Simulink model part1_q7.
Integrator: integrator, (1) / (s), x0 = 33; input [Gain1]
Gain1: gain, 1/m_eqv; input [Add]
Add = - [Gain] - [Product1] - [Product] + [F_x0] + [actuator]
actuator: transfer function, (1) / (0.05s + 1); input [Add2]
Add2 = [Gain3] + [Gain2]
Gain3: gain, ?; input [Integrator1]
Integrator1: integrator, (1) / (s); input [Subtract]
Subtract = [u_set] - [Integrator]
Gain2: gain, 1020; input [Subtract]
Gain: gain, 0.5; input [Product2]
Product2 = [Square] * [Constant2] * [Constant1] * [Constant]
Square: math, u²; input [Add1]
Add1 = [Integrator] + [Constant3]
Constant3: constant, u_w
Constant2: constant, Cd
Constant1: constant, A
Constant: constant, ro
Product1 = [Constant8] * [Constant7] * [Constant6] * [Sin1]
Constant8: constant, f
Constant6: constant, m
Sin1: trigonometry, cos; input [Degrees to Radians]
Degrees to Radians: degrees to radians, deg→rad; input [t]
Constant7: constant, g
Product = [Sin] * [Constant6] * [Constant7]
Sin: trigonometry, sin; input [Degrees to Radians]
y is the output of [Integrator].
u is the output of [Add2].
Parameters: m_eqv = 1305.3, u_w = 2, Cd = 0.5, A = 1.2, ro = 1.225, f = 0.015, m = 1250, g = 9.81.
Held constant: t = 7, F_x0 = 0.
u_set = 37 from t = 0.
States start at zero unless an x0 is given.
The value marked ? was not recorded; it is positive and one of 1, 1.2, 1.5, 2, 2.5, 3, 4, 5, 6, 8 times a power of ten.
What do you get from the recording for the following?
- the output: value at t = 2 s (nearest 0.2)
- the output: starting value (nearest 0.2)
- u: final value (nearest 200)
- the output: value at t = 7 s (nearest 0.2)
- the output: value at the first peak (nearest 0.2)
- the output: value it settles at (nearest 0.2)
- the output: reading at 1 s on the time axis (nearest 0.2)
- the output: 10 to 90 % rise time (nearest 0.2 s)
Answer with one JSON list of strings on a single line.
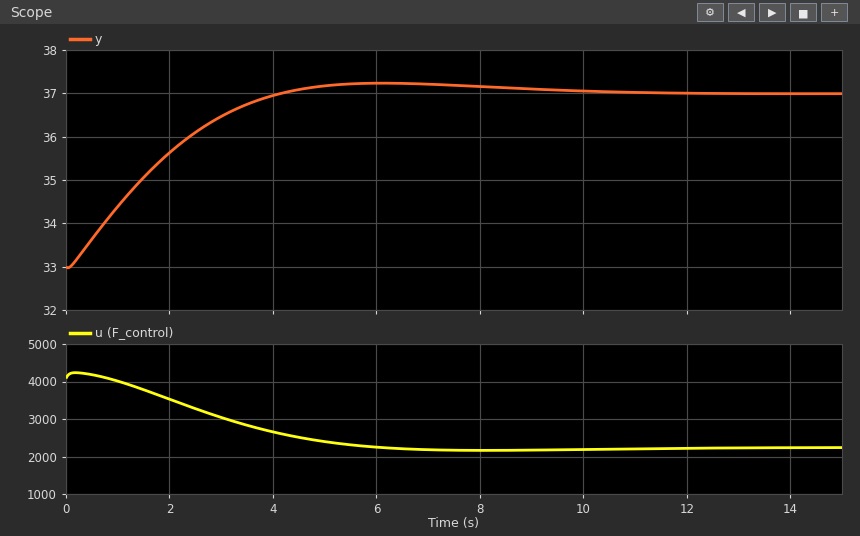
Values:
["35.6", "33.0", "2200", "37.2", "37.2", "37.0", "34.4", "2.8 s"]
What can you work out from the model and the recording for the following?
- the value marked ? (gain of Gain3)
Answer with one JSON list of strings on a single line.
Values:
["400"]
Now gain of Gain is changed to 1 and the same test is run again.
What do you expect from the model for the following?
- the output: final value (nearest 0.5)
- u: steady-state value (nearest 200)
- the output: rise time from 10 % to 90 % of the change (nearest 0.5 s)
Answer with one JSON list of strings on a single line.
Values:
["37.0", "2800", "3.5 s"]
